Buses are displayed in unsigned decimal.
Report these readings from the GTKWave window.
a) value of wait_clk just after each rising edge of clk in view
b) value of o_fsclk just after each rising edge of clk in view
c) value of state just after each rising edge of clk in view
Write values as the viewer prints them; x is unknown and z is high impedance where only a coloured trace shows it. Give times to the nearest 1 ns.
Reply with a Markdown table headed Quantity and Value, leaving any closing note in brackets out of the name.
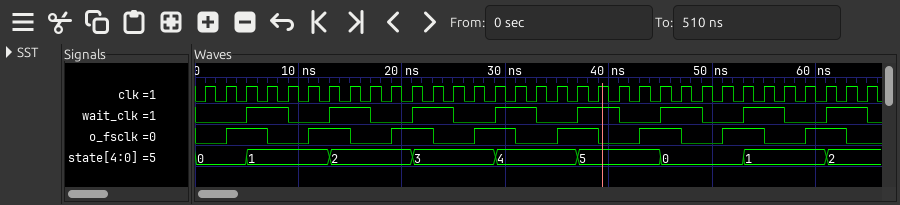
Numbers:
| Quantity | Value |
|---|---|
| value of wait_clk just after each rising edge of clk in view | 0 0 1 1 0 0 1 1 0 0 1 1 0 0 1 1 0 0 1 1 0 0 1 1 0 0 1 1 0 0 1 1 0 |
| value of o_fsclk just after each rising edge of clk in view | 0 1 1 0 0 1 1 0 0 1 1 0 0 1 1 0 0 1 1 0 0 1 1 0 0 1 1 0 0 1 1 0 0 |
| value of state just after each rising edge of clk in view | 0, 0, 1, 1, 1, 1, 2, 2, 2, 2, 3, 3, 3, 3, 4, 4, 4, 4, 5, 5, 5, 5, 0, 0, 0, 0, 1, 1, 1, 1, 2, 2, 2 |
